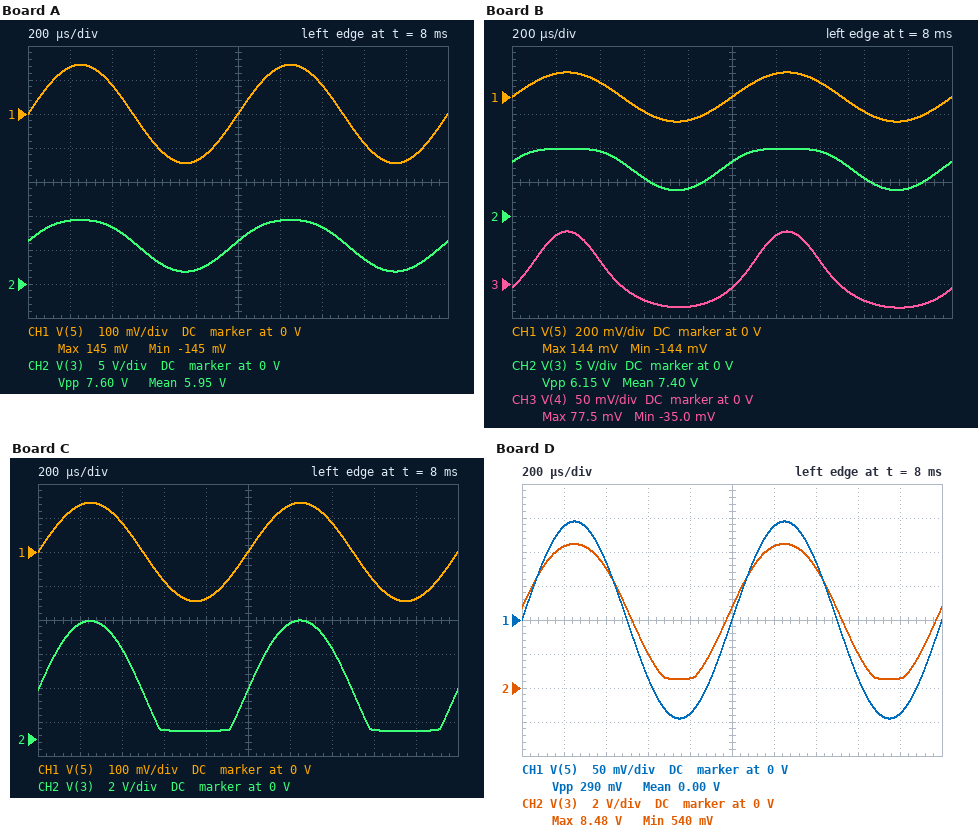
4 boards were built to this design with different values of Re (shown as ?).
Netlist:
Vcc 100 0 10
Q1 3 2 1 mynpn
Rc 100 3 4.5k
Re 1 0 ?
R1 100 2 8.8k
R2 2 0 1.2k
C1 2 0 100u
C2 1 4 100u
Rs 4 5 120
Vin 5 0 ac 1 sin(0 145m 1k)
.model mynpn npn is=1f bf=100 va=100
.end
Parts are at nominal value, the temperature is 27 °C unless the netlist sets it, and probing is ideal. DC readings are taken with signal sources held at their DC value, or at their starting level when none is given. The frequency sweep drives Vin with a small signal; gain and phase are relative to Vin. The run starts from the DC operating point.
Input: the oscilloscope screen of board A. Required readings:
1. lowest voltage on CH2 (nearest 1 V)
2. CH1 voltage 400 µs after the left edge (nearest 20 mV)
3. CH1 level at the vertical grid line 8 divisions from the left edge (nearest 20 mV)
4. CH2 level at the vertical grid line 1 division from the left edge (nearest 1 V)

2 V
80 mV
-80 mV
9 V
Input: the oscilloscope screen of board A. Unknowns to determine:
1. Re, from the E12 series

560 Ω
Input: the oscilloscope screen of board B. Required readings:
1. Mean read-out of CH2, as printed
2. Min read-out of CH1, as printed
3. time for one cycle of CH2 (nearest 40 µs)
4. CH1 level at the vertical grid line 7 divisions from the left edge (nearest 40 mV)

7.40 V
-144 mV
1.00 ms
80 mV
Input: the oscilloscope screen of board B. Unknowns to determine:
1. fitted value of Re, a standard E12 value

1 kΩ
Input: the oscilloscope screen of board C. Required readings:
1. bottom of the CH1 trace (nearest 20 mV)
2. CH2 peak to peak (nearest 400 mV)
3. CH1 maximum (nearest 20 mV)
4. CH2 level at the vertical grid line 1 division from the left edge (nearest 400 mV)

-140 mV
6.4 V
140 mV
6.8 V
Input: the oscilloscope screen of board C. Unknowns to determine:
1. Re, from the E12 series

270 Ω
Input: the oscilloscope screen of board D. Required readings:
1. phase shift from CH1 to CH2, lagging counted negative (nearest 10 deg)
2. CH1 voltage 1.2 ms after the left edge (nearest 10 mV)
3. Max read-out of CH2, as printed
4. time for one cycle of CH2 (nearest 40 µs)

0 deg
140 mV
8.48 V
1.00 ms
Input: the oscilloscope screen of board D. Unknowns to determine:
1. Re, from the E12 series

390 Ω
